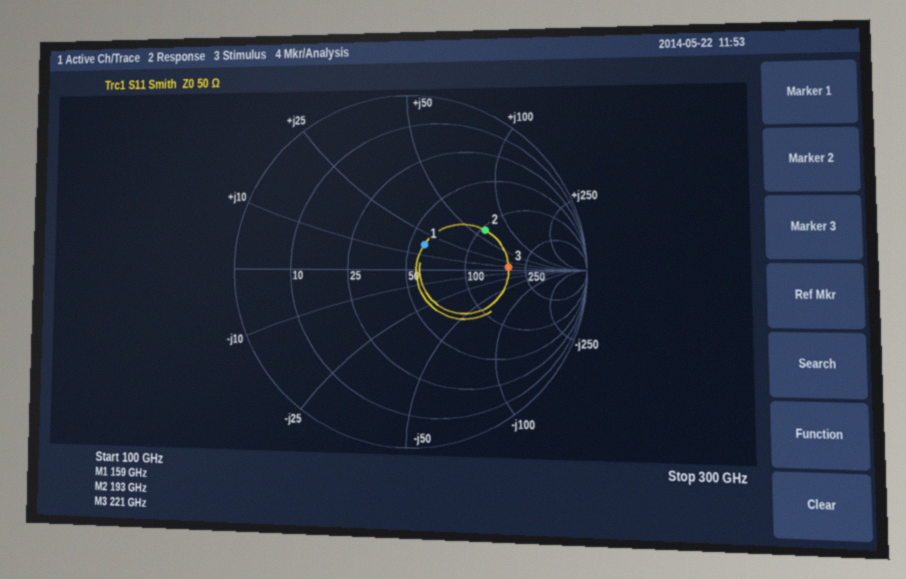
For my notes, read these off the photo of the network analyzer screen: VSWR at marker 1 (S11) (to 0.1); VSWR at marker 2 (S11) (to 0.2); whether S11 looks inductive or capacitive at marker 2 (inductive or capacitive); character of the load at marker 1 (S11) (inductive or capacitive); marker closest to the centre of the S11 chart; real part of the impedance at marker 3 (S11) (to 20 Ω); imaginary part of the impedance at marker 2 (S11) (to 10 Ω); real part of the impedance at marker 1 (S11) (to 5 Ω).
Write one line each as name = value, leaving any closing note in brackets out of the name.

VSWR at marker 1 (S11) = 1.4
VSWR at marker 2 (S11) = 3.0
whether S11 looks inductive or capacitive at marker 2 = inductive
character of the load at marker 1 (S11) = inductive
marker closest to the centre of the S11 chart = marker 1
real part of the impedance at marker 3 (S11) = 180 Ω
imaginary part of the impedance at marker 2 (S11) = +60 Ω
real part of the impedance at marker 1 (S11) = 60 Ω
